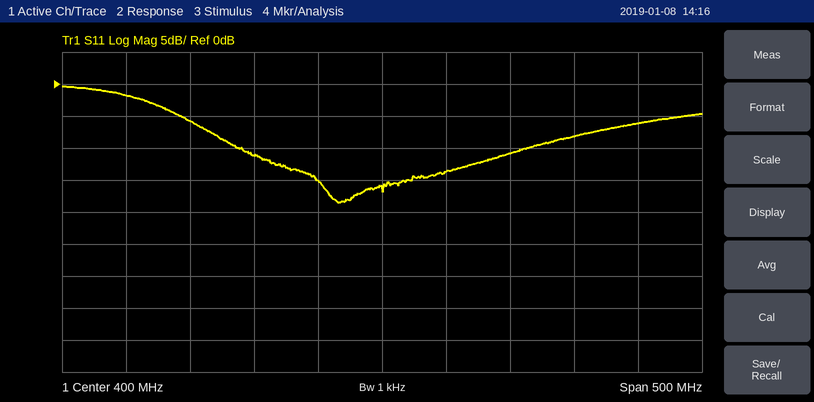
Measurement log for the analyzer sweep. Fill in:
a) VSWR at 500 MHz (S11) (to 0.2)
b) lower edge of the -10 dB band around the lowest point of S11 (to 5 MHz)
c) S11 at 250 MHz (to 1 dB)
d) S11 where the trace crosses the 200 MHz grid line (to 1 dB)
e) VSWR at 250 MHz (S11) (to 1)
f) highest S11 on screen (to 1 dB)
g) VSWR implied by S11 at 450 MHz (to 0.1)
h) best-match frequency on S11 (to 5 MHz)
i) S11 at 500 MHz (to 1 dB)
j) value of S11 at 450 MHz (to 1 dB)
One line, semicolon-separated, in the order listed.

1.8; 290 MHz; -6 dB; -2 dB; 3; 0 dB; 1.5; 365 MHz; -11 dB; -14 dB
